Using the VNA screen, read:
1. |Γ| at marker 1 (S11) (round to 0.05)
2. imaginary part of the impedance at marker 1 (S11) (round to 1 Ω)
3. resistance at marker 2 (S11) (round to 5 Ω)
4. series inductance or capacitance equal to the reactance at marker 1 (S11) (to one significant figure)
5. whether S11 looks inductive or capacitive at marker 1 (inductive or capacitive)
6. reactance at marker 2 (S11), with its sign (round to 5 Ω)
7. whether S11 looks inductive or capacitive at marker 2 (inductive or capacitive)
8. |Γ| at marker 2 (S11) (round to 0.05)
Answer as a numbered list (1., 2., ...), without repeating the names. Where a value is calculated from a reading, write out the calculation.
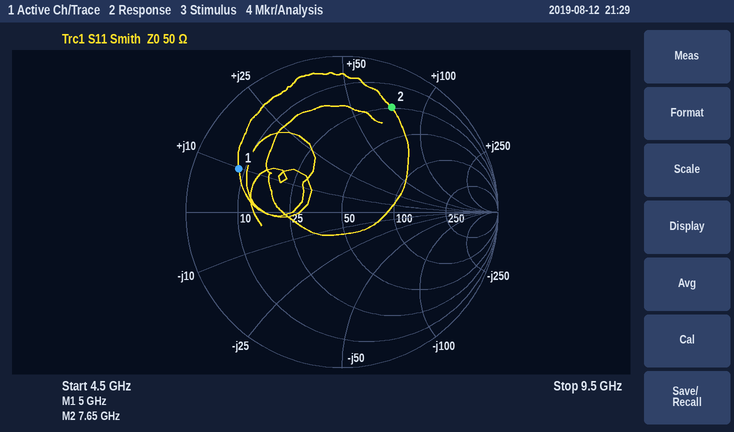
1. 0.70
2. +10 Ω
3. 25 Ω
4. L = 10 Ω/(2π × 5 GHz) ≈ 318 pH, so 300 pH to one significant figure
5. inductive
6. +75 Ω
7. inductive
8. 0.75
